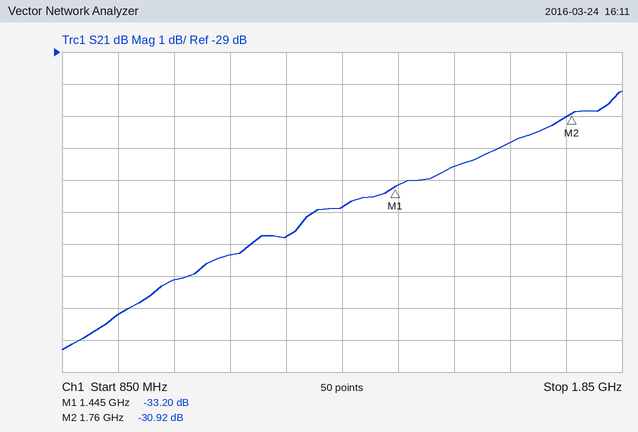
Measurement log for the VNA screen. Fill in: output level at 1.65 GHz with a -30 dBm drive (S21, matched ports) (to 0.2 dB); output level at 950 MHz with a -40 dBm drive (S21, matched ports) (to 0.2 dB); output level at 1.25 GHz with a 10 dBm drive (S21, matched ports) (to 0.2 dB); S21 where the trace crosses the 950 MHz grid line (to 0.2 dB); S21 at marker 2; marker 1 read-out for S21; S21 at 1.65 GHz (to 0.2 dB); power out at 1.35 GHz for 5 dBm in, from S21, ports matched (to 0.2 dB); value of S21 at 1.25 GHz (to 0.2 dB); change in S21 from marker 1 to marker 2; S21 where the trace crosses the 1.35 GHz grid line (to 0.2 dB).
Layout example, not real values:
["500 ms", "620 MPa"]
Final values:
["-61.8 dBm", "-77.2 dBm", "-24.8 dBm", "-37.2 dB", "-30.92 dB", "-33.20 dB", "-31.8 dB", "-28.8 dBm", "-34.8 dB", "2.28 dB", "-33.8 dB"]
